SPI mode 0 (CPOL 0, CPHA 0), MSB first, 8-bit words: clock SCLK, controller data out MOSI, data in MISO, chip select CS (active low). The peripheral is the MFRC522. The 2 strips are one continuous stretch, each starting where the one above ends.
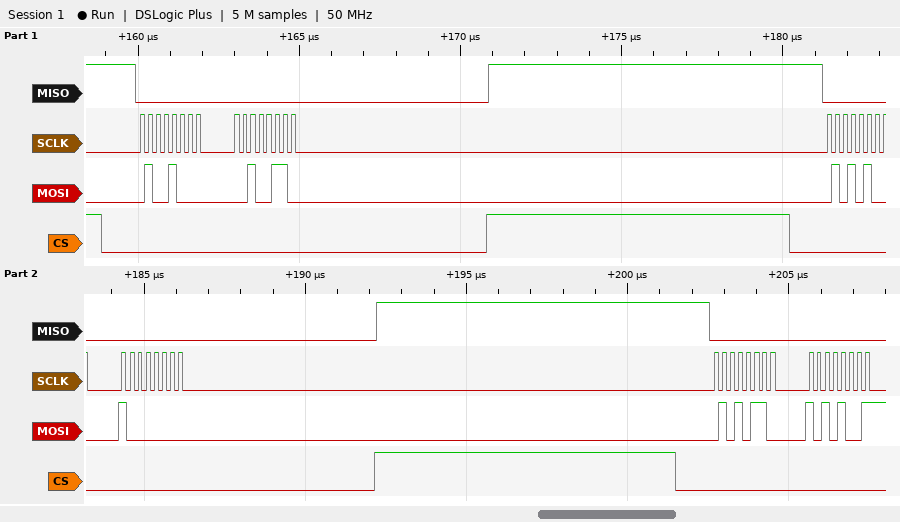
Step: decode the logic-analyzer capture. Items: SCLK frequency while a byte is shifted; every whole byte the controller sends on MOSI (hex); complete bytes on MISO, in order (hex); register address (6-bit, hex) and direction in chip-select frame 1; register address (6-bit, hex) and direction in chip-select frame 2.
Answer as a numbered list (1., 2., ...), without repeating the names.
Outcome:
1. 4 MHz
2. 0x48 0x26 0x54 0x80 0x56 0xA9
3. 0x00 0x00 0x00 0x00 0x00 0x00
4. 0x24 write
5. 0x2A write
